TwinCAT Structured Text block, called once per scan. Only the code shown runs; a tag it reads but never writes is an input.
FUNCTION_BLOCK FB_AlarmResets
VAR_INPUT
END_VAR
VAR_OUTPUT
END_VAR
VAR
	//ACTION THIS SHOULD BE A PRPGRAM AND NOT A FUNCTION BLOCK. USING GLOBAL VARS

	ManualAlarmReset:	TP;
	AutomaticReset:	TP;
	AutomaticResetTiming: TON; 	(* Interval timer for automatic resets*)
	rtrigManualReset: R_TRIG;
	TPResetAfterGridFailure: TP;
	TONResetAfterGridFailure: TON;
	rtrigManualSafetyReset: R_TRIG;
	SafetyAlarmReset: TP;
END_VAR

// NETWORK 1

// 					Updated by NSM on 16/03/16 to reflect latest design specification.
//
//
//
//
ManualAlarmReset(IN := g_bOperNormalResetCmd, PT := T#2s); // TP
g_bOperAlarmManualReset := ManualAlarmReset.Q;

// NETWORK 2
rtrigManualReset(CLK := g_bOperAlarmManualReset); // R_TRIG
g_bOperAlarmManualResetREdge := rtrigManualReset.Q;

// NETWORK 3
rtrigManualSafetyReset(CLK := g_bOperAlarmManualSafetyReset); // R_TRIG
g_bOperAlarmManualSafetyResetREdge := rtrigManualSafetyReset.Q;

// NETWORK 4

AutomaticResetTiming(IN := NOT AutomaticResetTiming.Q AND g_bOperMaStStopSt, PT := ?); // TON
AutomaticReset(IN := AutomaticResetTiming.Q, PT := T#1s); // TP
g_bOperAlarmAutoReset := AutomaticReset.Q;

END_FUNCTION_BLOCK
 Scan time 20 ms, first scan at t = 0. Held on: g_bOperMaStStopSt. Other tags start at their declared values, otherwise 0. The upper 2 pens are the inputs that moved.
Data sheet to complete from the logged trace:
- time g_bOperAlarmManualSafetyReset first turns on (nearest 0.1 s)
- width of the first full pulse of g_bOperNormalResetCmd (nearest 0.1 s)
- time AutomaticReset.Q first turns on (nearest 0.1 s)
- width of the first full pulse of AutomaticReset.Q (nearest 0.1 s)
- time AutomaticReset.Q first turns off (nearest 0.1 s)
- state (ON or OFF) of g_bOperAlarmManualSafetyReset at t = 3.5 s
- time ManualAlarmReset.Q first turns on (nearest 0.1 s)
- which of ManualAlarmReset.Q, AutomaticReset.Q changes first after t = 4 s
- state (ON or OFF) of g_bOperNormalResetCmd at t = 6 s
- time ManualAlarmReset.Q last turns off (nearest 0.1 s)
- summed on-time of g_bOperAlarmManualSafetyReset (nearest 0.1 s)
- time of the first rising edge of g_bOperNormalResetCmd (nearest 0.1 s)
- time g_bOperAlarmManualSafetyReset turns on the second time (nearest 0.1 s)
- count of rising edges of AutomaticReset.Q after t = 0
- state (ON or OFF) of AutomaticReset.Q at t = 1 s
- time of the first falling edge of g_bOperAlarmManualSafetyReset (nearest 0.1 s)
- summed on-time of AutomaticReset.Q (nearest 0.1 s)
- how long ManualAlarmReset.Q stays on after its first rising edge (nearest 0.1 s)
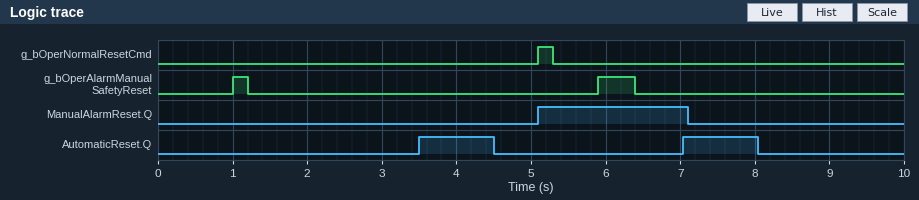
1.0 s
0.2 s
3.5 s
1.0 s
4.5 s
OFF
5.1 s
AutomaticReset.Q
OFF
7.1 s
0.7 s
5.1 s
5.9 s
2
OFF
1.2 s
2.0 s
2.0 s
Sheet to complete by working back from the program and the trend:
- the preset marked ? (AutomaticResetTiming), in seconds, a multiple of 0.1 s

3.5 s
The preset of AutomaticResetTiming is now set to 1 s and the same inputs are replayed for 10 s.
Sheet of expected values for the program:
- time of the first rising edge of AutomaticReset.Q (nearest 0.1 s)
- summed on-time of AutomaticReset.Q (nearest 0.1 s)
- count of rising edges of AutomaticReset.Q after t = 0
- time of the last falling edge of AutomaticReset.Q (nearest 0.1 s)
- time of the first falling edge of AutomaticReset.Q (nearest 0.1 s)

1.0 s
8.7 s
9
9.3 s
2.0 s
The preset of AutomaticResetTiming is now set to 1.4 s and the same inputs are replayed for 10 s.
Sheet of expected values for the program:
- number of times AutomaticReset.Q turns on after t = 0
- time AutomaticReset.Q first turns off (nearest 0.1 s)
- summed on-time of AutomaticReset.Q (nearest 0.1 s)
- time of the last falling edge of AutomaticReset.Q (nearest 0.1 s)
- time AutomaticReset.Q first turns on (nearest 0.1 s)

6
2.4 s
6.0 s
9.6 s
1.4 s
